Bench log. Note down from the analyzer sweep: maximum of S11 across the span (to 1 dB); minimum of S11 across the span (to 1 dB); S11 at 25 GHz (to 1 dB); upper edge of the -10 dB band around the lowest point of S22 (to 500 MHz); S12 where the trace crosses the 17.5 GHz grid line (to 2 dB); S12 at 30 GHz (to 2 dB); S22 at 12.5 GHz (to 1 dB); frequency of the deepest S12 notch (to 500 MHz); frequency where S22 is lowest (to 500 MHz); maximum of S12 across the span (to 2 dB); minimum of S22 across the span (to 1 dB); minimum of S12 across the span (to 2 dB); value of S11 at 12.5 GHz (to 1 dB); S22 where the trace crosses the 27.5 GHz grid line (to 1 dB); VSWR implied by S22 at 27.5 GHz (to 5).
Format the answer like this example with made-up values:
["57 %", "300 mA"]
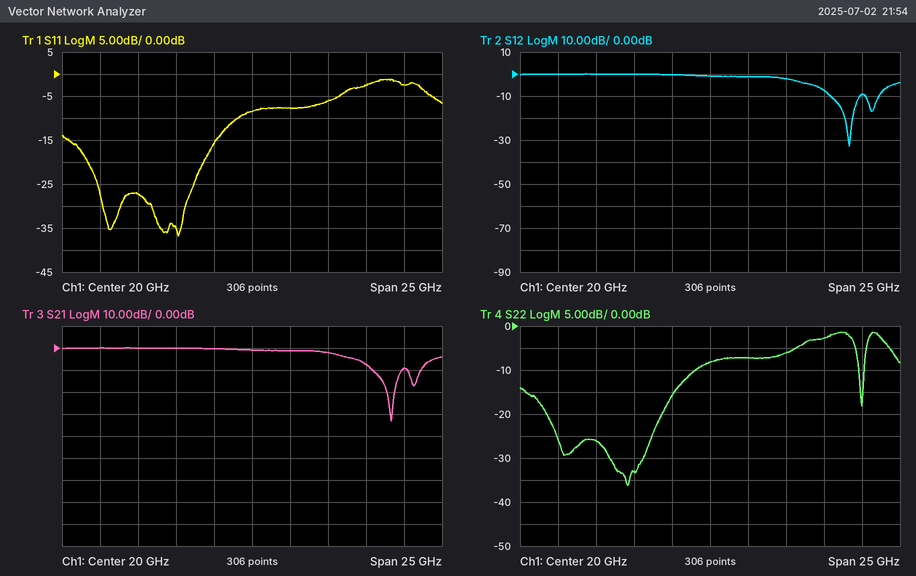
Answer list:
["-1 dB", "-37 dB", "-6 dB", "19.0 GHz", "0 dB", "-10 dB", "-26 dB", "29.0 GHz", "14.5 GHz", "0 dB", "-36 dB", "-32 dB", "-27 dB", "-3 dB", "5"]
